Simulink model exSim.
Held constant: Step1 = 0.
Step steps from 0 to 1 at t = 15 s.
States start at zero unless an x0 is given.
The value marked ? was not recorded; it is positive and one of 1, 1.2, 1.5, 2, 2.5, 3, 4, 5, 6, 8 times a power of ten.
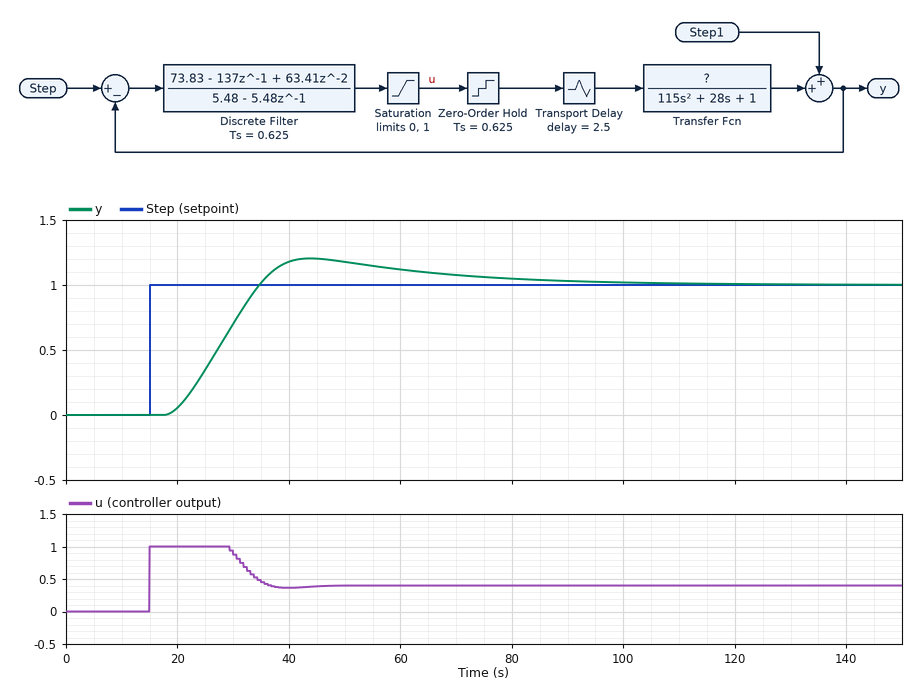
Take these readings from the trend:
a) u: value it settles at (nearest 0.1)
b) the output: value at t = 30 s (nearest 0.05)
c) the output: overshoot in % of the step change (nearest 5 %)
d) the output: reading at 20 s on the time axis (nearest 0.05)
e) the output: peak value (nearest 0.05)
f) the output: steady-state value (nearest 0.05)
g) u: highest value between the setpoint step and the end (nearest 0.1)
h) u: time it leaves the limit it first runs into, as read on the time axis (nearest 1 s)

0.4
0.70
20 %
0.05
1.20
1.00
1.0
29 s
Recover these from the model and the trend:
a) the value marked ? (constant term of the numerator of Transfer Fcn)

2.5
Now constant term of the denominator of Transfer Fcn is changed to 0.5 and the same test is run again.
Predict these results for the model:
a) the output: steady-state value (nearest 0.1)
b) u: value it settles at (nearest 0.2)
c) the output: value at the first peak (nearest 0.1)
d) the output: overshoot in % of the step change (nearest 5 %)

1.0
0.2
1.3
30 %
